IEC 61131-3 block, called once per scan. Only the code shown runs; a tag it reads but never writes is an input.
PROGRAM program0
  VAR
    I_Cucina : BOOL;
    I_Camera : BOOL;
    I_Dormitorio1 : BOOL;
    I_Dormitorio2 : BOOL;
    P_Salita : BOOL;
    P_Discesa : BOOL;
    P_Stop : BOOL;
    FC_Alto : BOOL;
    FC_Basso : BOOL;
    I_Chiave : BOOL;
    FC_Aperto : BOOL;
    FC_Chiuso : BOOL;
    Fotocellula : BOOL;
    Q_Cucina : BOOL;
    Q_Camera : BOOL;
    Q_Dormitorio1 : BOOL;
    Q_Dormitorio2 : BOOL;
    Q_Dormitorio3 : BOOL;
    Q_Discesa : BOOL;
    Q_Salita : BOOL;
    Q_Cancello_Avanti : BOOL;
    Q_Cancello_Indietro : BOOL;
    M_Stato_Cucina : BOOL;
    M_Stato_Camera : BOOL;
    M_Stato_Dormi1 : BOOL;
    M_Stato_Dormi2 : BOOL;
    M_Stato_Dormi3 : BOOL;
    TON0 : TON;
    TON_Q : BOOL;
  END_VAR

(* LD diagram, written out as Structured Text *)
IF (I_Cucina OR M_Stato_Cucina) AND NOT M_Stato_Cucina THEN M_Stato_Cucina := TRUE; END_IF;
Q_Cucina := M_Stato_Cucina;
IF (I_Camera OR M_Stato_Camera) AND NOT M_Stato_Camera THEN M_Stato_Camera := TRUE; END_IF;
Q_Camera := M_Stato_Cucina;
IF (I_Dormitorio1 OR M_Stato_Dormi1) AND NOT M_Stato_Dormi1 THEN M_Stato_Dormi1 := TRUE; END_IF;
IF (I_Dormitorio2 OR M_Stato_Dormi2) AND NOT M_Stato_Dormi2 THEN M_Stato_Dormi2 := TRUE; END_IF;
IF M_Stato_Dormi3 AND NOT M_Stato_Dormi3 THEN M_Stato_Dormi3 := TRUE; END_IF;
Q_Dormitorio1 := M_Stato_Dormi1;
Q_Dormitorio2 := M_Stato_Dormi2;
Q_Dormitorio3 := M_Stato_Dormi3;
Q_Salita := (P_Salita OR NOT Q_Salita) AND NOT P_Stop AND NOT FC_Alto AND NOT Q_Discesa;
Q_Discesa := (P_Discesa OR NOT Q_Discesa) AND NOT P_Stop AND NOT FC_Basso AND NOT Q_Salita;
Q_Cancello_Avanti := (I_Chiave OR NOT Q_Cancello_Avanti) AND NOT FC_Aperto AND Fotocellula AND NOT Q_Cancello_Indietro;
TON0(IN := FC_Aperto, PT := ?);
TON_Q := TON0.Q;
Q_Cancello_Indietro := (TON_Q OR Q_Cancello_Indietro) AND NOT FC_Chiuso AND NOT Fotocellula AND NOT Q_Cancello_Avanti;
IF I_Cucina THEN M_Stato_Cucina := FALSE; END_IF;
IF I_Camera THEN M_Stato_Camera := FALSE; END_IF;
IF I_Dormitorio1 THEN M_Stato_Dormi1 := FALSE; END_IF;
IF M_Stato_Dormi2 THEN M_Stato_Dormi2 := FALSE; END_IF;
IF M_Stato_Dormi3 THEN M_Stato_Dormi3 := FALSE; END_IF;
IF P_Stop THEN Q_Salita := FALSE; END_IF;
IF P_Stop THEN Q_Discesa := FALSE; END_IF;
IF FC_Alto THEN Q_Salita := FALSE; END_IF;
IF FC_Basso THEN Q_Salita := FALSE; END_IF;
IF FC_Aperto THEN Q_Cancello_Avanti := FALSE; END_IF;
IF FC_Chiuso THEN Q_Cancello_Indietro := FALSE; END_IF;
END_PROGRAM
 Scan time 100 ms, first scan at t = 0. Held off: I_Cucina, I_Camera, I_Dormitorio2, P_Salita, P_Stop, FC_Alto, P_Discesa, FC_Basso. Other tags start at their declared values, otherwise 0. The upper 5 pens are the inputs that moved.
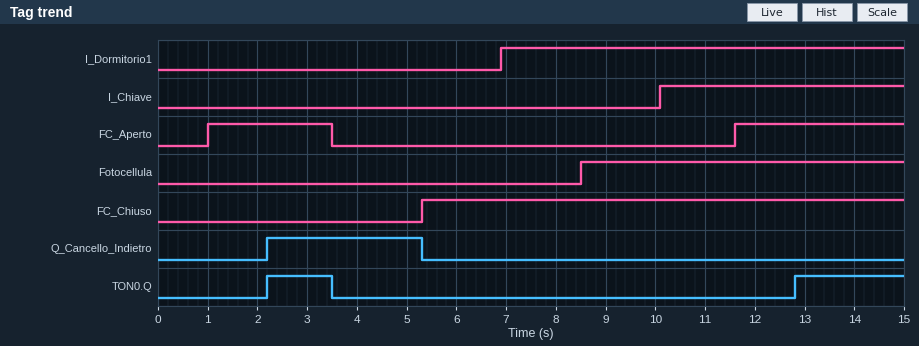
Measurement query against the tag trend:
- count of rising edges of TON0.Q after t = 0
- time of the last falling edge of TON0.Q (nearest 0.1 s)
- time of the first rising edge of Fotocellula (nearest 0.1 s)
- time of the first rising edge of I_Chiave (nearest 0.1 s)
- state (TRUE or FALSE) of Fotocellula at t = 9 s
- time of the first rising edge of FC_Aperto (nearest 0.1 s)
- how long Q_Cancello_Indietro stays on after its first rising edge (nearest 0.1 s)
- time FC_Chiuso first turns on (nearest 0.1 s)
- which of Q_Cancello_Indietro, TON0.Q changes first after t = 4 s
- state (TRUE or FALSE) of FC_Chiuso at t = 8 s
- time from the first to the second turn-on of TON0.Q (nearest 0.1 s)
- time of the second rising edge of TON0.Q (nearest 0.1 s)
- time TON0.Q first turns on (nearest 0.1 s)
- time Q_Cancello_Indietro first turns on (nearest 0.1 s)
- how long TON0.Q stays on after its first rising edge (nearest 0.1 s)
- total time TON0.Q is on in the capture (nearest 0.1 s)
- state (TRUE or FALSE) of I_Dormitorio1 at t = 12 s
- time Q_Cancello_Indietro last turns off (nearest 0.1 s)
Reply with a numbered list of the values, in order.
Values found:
1. 2
2. 3.5 s
3. 8.5 s
4. 10.1 s
5. TRUE
6. 1.0 s
7. 3.1 s
8. 5.3 s
9. Q_Cancello_Indietro
10. TRUE
11. 10.6 s
12. 12.8 s
13. 2.2 s
14. 2.2 s
15. 1.3 s
16. 3.5 s
17. TRUE
18. 5.3 s
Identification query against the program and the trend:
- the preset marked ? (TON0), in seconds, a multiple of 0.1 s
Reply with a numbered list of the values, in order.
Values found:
1. 1.2 s
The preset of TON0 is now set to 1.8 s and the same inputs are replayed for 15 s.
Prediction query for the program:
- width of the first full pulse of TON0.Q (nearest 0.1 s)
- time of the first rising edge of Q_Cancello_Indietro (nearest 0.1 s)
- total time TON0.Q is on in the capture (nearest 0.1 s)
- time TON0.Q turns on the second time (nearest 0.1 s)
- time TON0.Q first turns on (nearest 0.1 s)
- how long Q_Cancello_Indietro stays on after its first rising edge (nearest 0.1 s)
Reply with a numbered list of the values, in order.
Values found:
1. 0.7 s
2. 2.8 s
3. 2.3 s
4. 13.4 s
5. 2.8 s
6. 2.5 s
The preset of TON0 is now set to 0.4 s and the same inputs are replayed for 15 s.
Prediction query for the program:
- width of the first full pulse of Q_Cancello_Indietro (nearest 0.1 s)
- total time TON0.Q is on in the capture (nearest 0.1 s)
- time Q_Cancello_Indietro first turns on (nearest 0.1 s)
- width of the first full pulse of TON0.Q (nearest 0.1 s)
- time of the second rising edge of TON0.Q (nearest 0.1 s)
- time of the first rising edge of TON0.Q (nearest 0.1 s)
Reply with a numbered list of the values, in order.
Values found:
1. 3.9 s
2. 5.1 s
3. 1.4 s
4. 2.1 s
5. 12.0 s
6. 1.4 s
